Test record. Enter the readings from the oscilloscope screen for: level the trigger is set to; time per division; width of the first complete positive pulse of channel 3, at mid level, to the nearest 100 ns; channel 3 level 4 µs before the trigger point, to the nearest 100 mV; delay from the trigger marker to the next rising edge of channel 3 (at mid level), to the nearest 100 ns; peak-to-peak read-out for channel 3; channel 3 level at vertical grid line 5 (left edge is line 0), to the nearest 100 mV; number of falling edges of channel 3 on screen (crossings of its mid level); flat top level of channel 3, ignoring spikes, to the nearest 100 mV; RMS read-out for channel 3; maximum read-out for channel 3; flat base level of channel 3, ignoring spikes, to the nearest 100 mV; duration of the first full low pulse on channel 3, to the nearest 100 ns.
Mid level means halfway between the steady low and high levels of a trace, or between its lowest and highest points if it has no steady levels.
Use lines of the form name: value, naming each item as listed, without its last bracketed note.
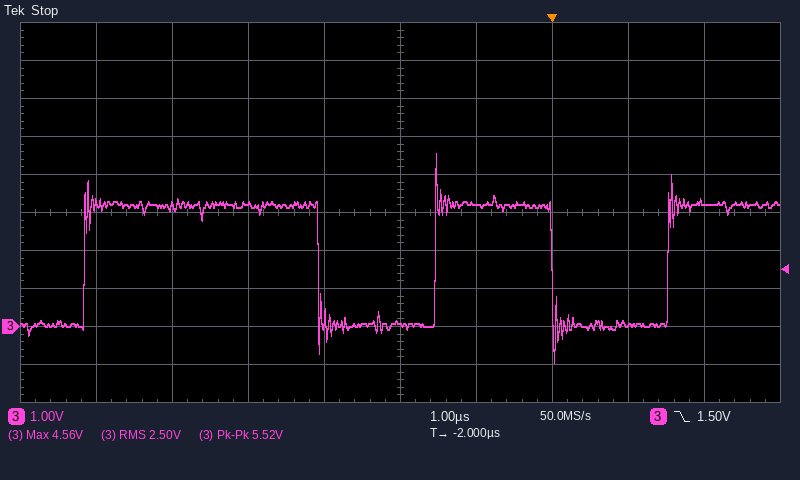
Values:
level the trigger is set to: 1.50 V
time per division: 1 µs
width of the first complete positive pulse of channel 3, at mid level, to the nearest 100 ns: 3.1 µs
channel 3 level 4 µs before the trigger point, to the nearest 100 mV: 3.2 V
delay from the trigger marker to the next rising edge of channel 3 (at mid level), to the nearest 100 ns: 1.5 µs
peak-to-peak read-out for channel 3: 5.52 V
channel 3 level at vertical grid line 5 (left edge is line 0), to the nearest 100 mV: 100 mV
number of falling edges of channel 3 on screen: 2
flat top level of channel 3, ignoring spikes, to the nearest 100 mV: 3.2 V
RMS read-out for channel 3: 2.50 V
maximum read-out for channel 3: 4.56 V
flat base level of channel 3, ignoring spikes, to the nearest 100 mV: 0.0 V
duration of the first full low pulse on channel 3, to the nearest 100 ns: 1.5 µs
